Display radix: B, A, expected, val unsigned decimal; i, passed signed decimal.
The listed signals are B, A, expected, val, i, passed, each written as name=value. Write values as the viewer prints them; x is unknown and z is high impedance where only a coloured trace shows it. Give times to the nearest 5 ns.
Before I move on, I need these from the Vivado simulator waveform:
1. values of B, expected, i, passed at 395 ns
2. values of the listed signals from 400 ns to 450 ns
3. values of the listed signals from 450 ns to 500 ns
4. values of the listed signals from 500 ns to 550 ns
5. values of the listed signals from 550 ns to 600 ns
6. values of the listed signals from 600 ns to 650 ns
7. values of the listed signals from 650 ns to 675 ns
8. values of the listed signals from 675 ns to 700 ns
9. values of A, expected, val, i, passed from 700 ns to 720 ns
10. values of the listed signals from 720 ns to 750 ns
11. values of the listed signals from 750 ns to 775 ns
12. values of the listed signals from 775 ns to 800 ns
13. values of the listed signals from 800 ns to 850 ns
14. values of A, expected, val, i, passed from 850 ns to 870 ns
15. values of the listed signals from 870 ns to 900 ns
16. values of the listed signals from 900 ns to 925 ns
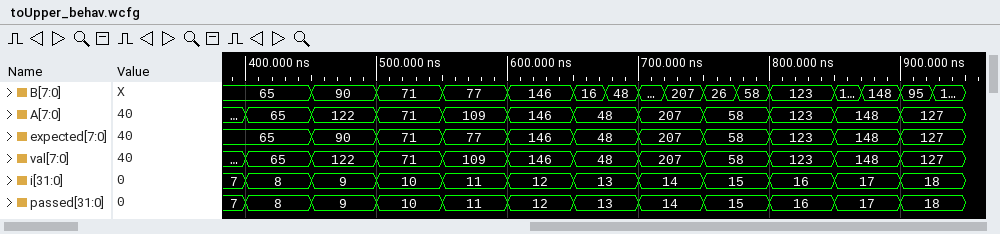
B=65, expected=65, i=7, passed=7
B=65, A=65, expected=65, val=65, i=8, passed=8
B=90, A=122, expected=90, val=122, i=9, passed=9
B=71, A=71, expected=71, val=71, i=10, passed=10
B=77, A=109, expected=77, val=109, i=11, passed=11
B=146, A=146, expected=146, val=146, i=12, passed=12
B=16, A=48, expected=48, val=48, i=13, passed=13
B=48, A=48, expected=48, val=48, i=13, passed=13
A=207, expected=207, val=207, i=14, passed=14
B=207, A=207, expected=207, val=207, i=14, passed=14
B=26, A=58, expected=58, val=58, i=15, passed=15
B=58, A=58, expected=58, val=58, i=15, passed=15
B=123, A=123, expected=123, val=123, i=16, passed=16
A=148, expected=148, val=148, i=17, passed=17
B=148, A=148, expected=148, val=148, i=17, passed=17
B=95, A=127, expected=127, val=127, i=18, passed=18
